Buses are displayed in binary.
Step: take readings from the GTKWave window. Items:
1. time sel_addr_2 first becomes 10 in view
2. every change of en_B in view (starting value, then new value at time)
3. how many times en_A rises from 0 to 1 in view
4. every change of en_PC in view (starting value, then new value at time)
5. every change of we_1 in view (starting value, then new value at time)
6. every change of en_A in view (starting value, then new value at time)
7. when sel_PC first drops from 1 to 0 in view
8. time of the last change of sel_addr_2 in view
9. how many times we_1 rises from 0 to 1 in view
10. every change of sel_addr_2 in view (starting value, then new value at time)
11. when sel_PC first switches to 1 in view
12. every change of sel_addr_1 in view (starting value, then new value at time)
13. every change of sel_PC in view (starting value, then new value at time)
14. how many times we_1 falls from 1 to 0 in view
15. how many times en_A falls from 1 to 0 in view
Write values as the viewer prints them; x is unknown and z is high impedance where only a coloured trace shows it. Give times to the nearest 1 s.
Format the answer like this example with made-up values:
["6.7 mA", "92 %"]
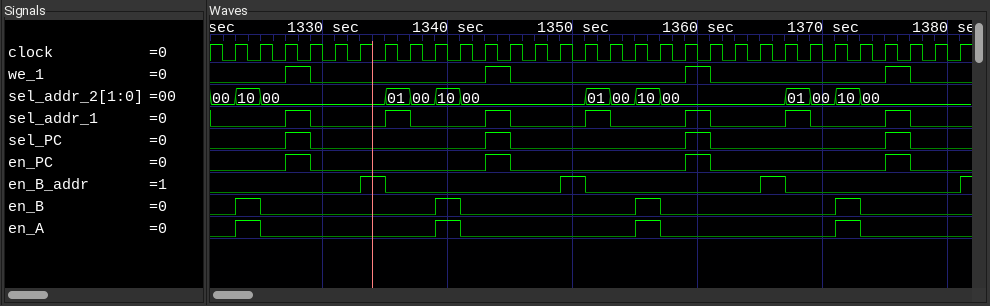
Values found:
["1323 s", "0, 1 at 1323 s, 0 at 1325 s, 1 at 1339 s, 0 at 1341 s, 1 at 1355 s, 0 at 1357 s, 1 at 1371 s, 0 at 1373 s", "4", "0, 1 at 1327 s, 0 at 1329 s, 1 at 1343 s, 0 at 1345 s, 1 at 1359 s, 0 at 1361 s, 1 at 1375 s, 0 at 1377 s", "0, 1 at 1327 s, 0 at 1329 s, 1 at 1343 s, 0 at 1345 s, 1 at 1359 s, 0 at 1361 s, 1 at 1375 s, 0 at 1377 s", "0, 1 at 1323 s, 0 at 1325 s, 1 at 1339 s, 0 at 1341 s, 1 at 1355 s, 0 at 1357 s, 1 at 1371 s, 0 at 1373 s", "1329 s", "1373 s", "4", "00, 10 at 1323 s, 00 at 1325 s, 01 at 1335 s, 00 at 1337 s, 10 at 1339 s, 00 at 1341 s, 01 at 1351 s, 00 at 1353 s, 10 at 1355 s, 00 at 1357 s, 01 at 1367 s, 00 at 1369 s, 10 at 1371 s, 00 at 1373 s", "1327 s", "0, 1 at 1327 s, 0 at 1329 s, 1 at 1335 s, 0 at 1337 s, 1 at 1343 s, 0 at 1345 s, 1 at 1351 s, 0 at 1353 s, 1 at 1359 s, 0 at 1361 s, 1 at 1367 s, 0 at 1369 s, 1 at 1375 s, 0 at 1377 s", "0, 1 at 1327 s, 0 at 1329 s, 1 at 1343 s, 0 at 1345 s, 1 at 1359 s, 0 at 1361 s, 1 at 1375 s, 0 at 1377 s", "4", "4"]
